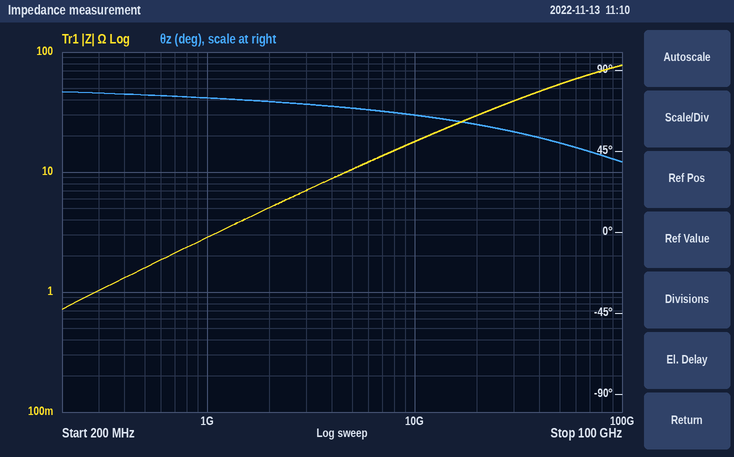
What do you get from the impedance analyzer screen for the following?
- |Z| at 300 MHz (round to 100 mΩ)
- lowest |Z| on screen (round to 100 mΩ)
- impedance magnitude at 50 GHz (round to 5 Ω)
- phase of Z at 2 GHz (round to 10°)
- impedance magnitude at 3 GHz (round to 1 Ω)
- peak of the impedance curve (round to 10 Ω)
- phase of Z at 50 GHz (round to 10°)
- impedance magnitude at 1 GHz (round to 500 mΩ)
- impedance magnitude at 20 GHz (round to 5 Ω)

1.0 Ω
700 mΩ
55 Ω
70°
7 Ω
80 Ω
50°
3.0 Ω
30 Ω
